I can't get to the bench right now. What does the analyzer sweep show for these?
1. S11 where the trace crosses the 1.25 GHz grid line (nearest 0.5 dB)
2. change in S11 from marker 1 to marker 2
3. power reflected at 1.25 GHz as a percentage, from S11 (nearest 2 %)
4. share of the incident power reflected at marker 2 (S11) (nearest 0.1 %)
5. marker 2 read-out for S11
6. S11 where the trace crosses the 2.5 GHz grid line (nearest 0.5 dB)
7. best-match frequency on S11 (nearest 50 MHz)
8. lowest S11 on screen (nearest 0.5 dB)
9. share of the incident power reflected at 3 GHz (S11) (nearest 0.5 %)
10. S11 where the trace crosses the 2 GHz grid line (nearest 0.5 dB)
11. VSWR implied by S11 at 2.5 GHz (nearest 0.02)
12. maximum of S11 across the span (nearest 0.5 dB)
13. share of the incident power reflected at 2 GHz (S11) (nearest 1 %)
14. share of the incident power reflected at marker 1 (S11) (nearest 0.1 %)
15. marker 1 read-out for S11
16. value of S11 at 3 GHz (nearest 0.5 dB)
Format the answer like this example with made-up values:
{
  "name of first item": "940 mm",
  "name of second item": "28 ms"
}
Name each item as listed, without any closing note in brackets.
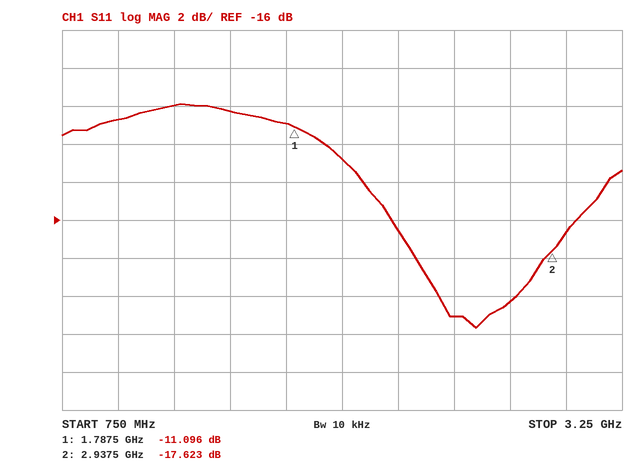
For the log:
{
  "S11 where the trace crosses the 1.25 GHz grid line": "-10.0 dB",
  "change in S11 from marker 1 to marker 2": "-6.527 dB",
  "power reflected at 1.25 GHz as a percentage, from S11": "10 %",
  "share of the incident power reflected at marker 2 (S11)": "1.7 %",
  "marker 2 read-out for S11": "-17.623 dB",
  "S11 where the trace crosses the 2.5 GHz grid line": "-21.0 dB",
  "best-match frequency on S11": "2.60 GHz",
  "lowest S11 on screen": "-21.5 dB",
  "share of the incident power reflected at 3 GHz (S11)": "2.0 %",
  "S11 where the trace crosses the 2 GHz grid line": "-13.0 dB",
  "VSWR implied by S11 at 2.5 GHz": "1.20",
  "maximum of S11 across the span": "-10.0 dB",
  "share of the incident power reflected at 2 GHz (S11)": "5 %",
  "share of the incident power reflected at marker 1 (S11)": "7.8 %",
  "marker 1 read-out for S11": "-11.096 dB",
  "value of S11 at 3 GHz": "-16.5 dB"
}
